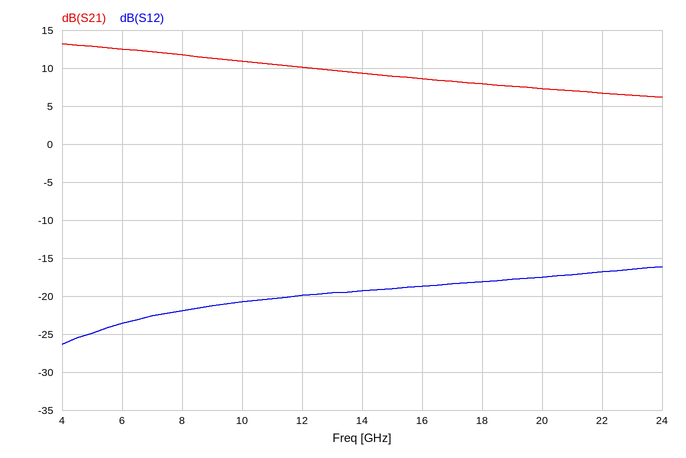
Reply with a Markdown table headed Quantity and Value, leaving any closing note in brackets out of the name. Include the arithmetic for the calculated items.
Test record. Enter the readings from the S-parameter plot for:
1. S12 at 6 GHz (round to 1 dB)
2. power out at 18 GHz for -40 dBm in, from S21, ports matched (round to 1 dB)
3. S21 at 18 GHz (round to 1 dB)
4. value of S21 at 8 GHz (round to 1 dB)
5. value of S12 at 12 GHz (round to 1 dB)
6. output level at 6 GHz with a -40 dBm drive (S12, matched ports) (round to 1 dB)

| Quantity | Value |
|---|---|
| S12 at 6 GHz | -24 dB |
| power out at 18 GHz for -40 dBm in, from S21, ports matched | -40 dBm + (8 dB) = -32 dBm |
| S21 at 18 GHz | 8 dB |
| value of S21 at 8 GHz | 12 dB |
| value of S12 at 12 GHz | -20 dB |
| output level at 6 GHz with a -40 dBm drive (S12, matched ports) | -40 dBm + (-24 dB) = -64 dBm |
